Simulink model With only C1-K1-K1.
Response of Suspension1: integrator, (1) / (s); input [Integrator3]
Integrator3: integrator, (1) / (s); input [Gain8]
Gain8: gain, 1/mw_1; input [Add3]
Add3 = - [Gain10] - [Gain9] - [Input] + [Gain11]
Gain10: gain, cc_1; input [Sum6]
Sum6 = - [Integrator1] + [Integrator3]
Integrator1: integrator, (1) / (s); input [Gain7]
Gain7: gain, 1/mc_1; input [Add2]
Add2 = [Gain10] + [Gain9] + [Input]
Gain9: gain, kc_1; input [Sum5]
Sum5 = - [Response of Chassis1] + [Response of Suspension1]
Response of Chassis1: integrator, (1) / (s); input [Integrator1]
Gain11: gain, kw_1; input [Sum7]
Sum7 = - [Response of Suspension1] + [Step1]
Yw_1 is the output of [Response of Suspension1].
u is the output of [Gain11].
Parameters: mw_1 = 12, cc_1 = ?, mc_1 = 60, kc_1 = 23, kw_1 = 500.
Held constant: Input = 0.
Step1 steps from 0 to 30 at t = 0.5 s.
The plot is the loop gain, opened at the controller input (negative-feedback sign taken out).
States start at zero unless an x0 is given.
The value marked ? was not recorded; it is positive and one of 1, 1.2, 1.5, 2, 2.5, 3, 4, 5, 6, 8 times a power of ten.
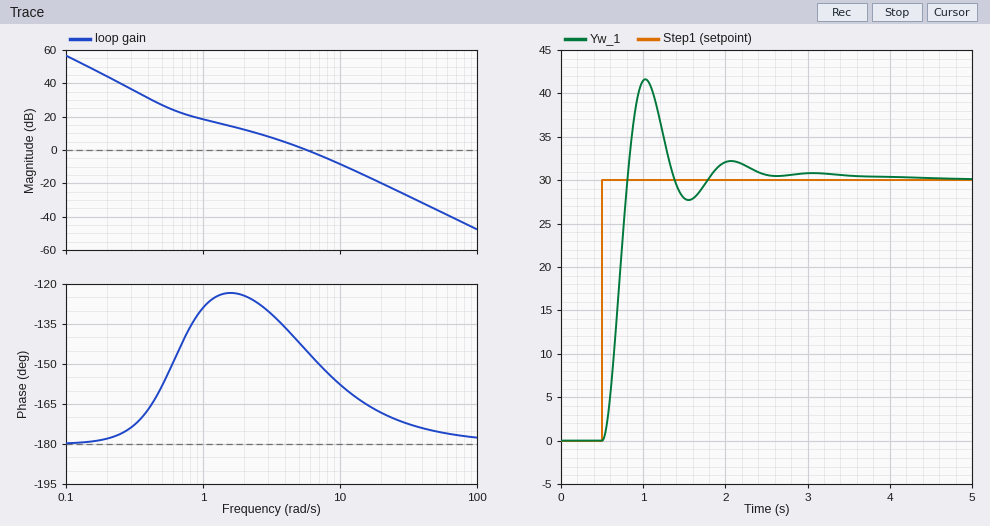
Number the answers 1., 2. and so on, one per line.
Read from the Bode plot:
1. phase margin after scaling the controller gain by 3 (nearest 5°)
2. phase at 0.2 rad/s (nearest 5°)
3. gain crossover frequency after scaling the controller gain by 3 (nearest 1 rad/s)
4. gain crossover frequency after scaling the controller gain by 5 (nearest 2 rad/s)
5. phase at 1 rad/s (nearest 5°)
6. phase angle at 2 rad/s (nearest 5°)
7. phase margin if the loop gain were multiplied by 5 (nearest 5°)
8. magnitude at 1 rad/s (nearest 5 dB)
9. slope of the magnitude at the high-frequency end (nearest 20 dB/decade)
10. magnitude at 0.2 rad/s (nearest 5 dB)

1. 20°
2. -180°
3. 11 rad/s
4. 14 rad/s
5. -130°
6. -125°
7. 15°
8. 20 dB
9. -40 dB/decade
10. 45 dB
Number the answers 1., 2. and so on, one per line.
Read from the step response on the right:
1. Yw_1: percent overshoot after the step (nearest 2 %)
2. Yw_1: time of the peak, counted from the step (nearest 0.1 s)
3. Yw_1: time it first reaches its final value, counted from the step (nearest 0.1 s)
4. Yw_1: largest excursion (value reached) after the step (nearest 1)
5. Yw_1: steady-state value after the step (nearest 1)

1. 38 %
2. 0.5 s
3. 0.3 s
4. 42
5. 30
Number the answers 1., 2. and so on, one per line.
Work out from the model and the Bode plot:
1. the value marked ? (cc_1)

1. 50
